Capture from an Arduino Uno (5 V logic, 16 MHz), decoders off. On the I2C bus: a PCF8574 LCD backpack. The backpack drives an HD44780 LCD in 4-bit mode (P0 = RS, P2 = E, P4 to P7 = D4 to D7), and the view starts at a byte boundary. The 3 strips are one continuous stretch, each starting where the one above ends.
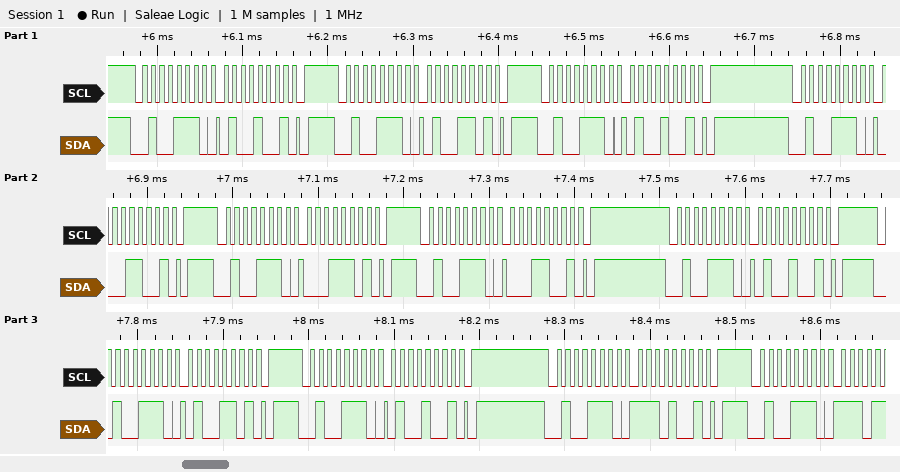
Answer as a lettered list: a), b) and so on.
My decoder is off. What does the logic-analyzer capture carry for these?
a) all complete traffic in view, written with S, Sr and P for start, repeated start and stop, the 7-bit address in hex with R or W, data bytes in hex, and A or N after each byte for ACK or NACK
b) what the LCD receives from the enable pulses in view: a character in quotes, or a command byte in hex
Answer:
a) S 27W A 49 A P S 27W A 4D A P S 27W A 49 A P S 27W A 19 A P S 27W A 1D A P S 27W A 19 A P S 27W A 49 A P S 27W A 4D A P S 27W A 49 A P S 27W A E9 A P S 27W A
b) 'A'
